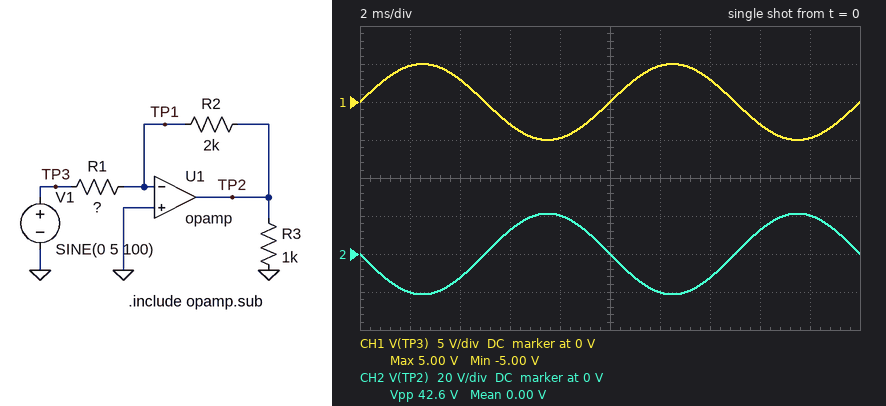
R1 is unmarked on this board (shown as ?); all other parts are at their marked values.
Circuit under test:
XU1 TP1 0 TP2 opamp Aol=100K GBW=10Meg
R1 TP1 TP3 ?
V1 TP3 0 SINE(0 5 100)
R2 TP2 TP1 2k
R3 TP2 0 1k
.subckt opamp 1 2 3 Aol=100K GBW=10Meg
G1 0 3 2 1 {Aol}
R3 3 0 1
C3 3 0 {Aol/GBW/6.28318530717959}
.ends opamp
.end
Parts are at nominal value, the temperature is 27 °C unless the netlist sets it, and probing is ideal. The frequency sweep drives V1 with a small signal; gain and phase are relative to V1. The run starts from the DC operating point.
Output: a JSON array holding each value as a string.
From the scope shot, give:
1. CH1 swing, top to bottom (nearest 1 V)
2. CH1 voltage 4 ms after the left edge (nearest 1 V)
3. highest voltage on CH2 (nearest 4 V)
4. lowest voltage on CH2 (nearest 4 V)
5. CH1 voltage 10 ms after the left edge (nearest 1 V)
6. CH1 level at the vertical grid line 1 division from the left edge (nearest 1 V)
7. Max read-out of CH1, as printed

["10 V", "3 V", "20 V", "-20 V", "0 V", "5 V", "5.00 V"]
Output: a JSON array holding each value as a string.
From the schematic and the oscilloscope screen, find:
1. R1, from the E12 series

["470 Ω"]
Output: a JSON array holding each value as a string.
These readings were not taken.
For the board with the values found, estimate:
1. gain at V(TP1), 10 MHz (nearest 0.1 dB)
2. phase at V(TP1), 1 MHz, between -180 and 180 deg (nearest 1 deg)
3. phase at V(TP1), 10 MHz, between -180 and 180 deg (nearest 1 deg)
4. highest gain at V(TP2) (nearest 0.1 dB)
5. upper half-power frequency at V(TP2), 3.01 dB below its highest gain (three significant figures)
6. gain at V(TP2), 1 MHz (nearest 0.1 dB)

["-2.0 dB", "62 deg", "11 deg", "12.6 dB", "1.90 MHz", "11.5 dB"]
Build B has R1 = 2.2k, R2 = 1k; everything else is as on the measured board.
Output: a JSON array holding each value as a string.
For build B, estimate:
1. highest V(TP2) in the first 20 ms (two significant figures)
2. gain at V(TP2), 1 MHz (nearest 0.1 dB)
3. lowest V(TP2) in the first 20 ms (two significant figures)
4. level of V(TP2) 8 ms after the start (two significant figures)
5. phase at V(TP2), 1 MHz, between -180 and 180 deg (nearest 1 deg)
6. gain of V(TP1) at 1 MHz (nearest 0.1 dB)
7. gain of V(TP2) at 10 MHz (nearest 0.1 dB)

["2.3 V", "-6.9 dB", "-2.3 V", "2.2 V", "172 deg", "-26.9 dB", "-11.8 dB"]
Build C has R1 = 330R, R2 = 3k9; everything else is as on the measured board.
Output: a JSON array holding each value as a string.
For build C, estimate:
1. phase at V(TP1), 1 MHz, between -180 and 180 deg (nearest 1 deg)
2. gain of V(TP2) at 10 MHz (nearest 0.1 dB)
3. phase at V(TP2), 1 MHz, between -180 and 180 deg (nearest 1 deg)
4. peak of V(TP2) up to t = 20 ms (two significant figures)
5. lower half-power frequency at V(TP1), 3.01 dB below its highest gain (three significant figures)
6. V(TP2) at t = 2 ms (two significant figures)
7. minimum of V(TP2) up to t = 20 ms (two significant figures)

["38 deg", "-0.7 dB", "128 deg", "59 V", "780 kHz", "-56 V", "-59 V"]
